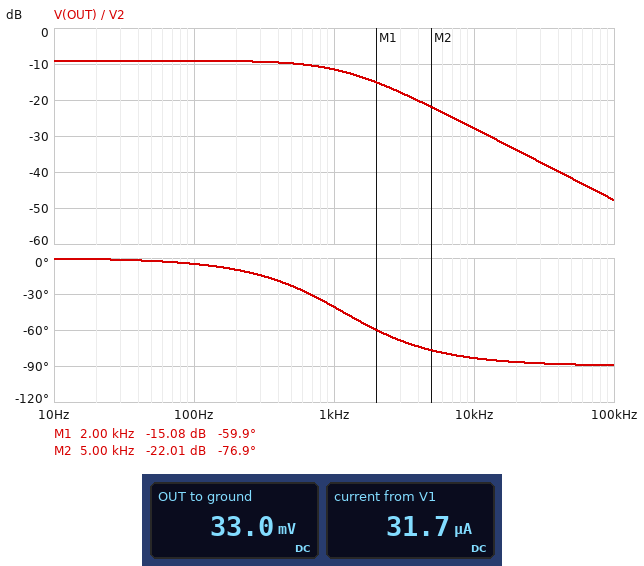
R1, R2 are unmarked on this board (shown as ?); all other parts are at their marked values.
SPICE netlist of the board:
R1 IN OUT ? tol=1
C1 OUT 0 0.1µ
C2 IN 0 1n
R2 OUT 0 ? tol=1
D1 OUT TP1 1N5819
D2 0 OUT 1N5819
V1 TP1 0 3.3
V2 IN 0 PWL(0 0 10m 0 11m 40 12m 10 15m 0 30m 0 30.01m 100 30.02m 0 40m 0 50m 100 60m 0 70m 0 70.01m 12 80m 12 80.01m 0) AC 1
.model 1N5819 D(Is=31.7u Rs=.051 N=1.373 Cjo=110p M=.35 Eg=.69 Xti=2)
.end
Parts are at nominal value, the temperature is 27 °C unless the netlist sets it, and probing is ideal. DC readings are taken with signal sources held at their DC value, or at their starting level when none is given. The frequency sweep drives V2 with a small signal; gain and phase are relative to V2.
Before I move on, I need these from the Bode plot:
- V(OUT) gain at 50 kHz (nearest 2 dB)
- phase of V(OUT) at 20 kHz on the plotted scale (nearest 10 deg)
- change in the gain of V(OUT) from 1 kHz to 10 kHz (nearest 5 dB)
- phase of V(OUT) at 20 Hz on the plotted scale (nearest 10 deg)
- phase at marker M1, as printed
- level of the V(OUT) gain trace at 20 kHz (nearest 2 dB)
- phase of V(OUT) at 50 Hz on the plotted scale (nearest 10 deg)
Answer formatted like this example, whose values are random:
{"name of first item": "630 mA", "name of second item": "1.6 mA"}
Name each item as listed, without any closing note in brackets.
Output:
{"V(OUT) gain at 50 kHz": "-42 dB", "phase of V(OUT) at 20 kHz on the plotted scale": "-90 deg", "change in the gain of V(OUT) from 1 kHz to 10 kHz": "-15 dB", "phase of V(OUT) at 20 Hz on the plotted scale": "0 deg", "phase at marker M1, as printed": "-59.9 deg", "level of the V(OUT) gain trace at 20 kHz": "-34 dB", "phase of V(OUT) at 50 Hz on the plotted scale": "0 deg"}
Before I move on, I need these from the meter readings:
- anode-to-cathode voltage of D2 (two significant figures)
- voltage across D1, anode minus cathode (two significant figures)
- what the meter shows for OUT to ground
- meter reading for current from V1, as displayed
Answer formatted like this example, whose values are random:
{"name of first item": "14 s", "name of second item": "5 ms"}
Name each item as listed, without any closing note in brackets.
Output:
{"anode-to-cathode voltage of D2": "-33 mV", "voltage across D1, anode minus cathode": "-3.3 V", "what the meter shows for OUT to ground": "33.0 mV", "meter reading for current from V1, as displayed": "31.7 µA"}
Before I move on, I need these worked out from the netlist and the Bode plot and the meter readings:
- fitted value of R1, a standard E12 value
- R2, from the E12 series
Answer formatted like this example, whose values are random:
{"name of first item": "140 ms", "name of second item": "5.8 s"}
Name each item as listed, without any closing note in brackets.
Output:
{"fitted value of R1, a standard E12 value": "3.9 kΩ", "R2, from the E12 series": "8.2 kΩ"}
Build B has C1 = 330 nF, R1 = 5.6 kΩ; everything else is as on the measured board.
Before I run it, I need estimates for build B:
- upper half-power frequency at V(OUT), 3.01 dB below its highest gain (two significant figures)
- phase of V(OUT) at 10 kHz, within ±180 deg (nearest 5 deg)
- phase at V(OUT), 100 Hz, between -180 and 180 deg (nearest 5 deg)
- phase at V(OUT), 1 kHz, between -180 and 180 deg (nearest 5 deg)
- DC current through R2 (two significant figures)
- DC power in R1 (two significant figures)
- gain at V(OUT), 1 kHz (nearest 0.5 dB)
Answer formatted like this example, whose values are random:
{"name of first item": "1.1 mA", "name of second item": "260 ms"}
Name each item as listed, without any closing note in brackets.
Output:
{"upper half-power frequency at V(OUT), 3.01 dB below its highest gain": "300 Hz", "phase of V(OUT) at 10 kHz, within ±180 deg": "-90 deg", "phase at V(OUT), 100 Hz, between -180 and 180 deg": "-20 deg", "phase at V(OUT), 1 kHz, between -180 and 180 deg": "-75 deg", "DC current through R2": "4.5 µA", "DC power in R1": "250 nW", "gain at V(OUT), 1 kHz": "-21.5 dB"}
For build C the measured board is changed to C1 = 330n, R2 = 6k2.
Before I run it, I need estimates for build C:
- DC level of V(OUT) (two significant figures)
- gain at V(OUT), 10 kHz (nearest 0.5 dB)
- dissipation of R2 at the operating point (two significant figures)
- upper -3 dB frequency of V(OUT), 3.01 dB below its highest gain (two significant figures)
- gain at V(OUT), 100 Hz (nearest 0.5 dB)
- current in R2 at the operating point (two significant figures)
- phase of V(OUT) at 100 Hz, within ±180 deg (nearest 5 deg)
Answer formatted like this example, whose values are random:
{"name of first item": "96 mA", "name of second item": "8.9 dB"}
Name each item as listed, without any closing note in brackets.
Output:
{"DC level of V(OUT)": "31 mV", "gain at V(OUT), 10 kHz": "-38.0 dB", "dissipation of R2 at the operating point": "160 nW", "upper -3 dB frequency of V(OUT), 3.01 dB below its highest gain": "380 Hz", "gain at V(OUT), 100 Hz": "-10.0 dB", "current in R2 at the operating point": "5.1 µA", "phase of V(OUT) at 100 Hz, within ±180 deg": "-15 deg"}
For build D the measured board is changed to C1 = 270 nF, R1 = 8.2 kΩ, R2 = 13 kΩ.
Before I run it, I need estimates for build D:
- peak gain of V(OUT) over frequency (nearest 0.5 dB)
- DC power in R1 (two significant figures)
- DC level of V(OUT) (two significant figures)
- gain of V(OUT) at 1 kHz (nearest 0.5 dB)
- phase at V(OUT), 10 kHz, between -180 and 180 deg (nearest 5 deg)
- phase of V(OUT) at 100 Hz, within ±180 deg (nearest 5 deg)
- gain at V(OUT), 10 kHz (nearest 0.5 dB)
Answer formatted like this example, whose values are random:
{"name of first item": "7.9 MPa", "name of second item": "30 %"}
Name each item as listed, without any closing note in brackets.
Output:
{"peak gain of V(OUT) over frequency": "-11.5 dB", "DC power in R1": "250 nW", "DC level of V(OUT)": "45 mV", "gain of V(OUT) at 1 kHz": "-23.0 dB", "phase at V(OUT), 10 kHz, between -180 and 180 deg": "-90 deg", "phase of V(OUT) at 100 Hz, within ±180 deg": "-20 deg", "gain at V(OUT), 10 kHz": "-43.0 dB"}
